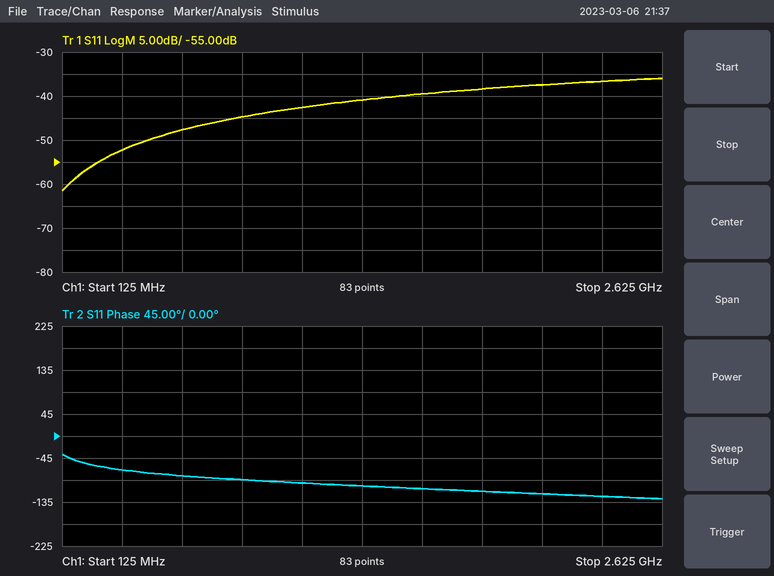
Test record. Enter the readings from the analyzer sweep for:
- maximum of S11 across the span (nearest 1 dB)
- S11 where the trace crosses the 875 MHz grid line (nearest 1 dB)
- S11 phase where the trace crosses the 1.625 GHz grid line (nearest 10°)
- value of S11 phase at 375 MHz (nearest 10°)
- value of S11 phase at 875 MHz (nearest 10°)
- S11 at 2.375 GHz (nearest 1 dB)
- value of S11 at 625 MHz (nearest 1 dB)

-36 dB
-45 dB
-110°
-70°
-90°
-37 dB
-48 dB
